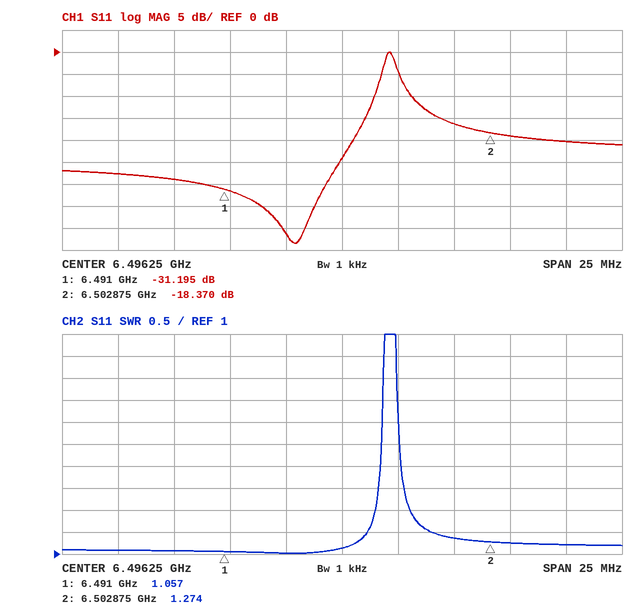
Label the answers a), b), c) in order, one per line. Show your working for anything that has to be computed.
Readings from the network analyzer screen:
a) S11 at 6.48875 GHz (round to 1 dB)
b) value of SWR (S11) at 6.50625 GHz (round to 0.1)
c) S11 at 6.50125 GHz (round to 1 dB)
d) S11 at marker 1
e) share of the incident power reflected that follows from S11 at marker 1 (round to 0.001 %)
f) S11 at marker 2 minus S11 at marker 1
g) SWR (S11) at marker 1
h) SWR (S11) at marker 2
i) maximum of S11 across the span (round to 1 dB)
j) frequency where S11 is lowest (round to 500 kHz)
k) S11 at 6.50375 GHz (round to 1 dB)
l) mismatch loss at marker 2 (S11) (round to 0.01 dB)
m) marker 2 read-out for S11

a) -29 dB
b) 1.2
c) -16 dB
d) -31.195 dB
e) 10^(-31.195/10) ≈ 0.076 %
f) -18.37 − (-31.195) = 12.825 dB
g) 1.057
h) 1.274
i) 0 dB
j) 6.4940 GHz
k) -19 dB
l) −10 log10(1 − 10^(-18.37/10)) ≈ 0.06 dB
m) -18.370 dB
